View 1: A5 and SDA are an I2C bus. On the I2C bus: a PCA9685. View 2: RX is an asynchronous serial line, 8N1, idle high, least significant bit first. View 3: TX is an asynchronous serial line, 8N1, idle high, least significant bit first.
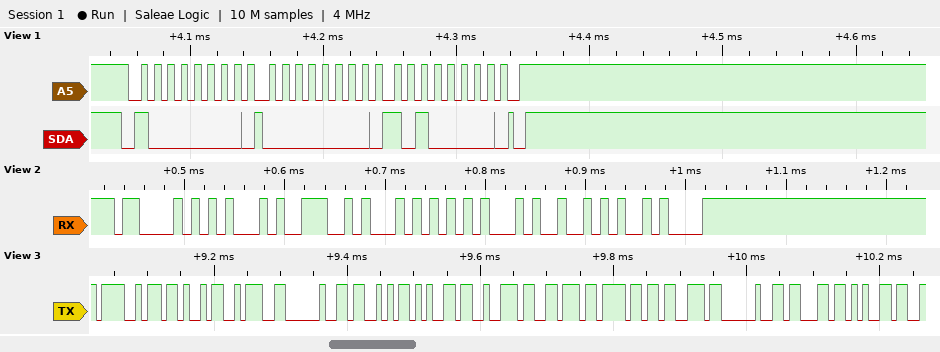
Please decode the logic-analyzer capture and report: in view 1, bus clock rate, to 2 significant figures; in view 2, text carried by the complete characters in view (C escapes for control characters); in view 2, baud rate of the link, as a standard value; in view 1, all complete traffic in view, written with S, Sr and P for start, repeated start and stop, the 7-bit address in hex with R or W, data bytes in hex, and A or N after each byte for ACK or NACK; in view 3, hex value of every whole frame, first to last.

100 kHz
"CENTER\n"
115200 baud
S 40W A 00 A A0 A P
4F 4B 3A 20 53 65 72 76 6F 73 20 63 65
